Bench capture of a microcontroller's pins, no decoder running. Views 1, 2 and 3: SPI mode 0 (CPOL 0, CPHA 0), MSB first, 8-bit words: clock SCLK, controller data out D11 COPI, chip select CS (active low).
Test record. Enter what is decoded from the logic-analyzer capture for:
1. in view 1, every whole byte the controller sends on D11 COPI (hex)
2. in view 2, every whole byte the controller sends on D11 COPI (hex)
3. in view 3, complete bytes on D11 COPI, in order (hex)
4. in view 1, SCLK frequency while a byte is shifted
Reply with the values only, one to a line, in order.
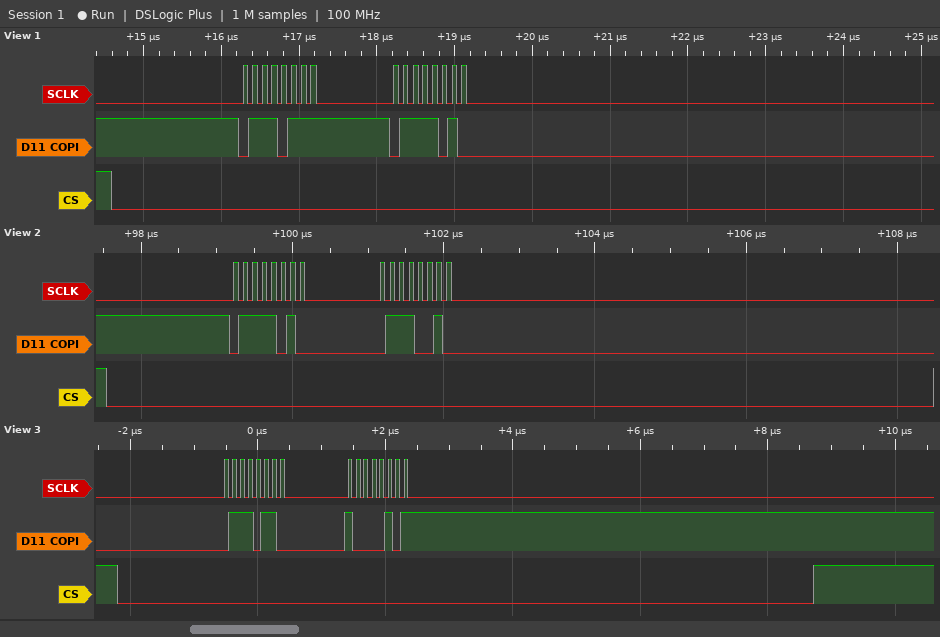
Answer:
77 7A
7A 72
76 85
8 MHz
